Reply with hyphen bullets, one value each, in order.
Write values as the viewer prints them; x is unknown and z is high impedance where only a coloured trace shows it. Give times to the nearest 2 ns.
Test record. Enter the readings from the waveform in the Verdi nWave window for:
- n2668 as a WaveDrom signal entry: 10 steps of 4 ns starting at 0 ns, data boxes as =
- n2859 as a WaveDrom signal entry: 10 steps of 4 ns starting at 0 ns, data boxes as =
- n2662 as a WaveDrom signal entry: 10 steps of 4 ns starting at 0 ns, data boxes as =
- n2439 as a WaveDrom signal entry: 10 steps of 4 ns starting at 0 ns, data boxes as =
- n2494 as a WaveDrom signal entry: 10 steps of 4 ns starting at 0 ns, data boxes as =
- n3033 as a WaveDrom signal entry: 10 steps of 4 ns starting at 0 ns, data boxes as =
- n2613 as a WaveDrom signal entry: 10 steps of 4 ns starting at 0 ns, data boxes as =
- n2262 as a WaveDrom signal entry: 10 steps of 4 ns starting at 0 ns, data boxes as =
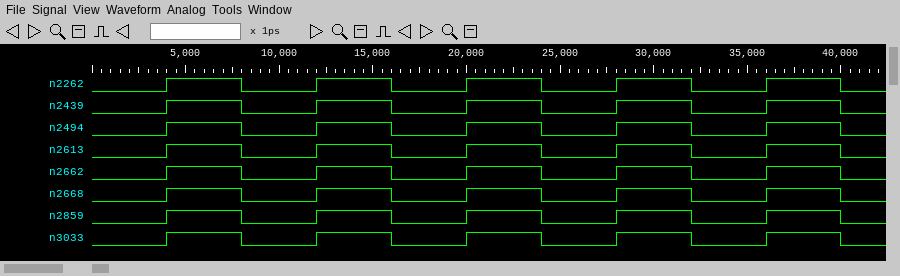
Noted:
- {name: 'n2668', wave: '0101010101'}
- {name: 'n2859', wave: '0101010101'}
- {name: 'n2662', wave: '0101010101'}
- {name: 'n2439', wave: '0101010101'}
- {name: 'n2494', wave: '0101010101'}
- {name: 'n3033', wave: '0101010101'}
- {name: 'n2613', wave: '0101010101'}
- {name: 'n2262', wave: '0101010101'}
